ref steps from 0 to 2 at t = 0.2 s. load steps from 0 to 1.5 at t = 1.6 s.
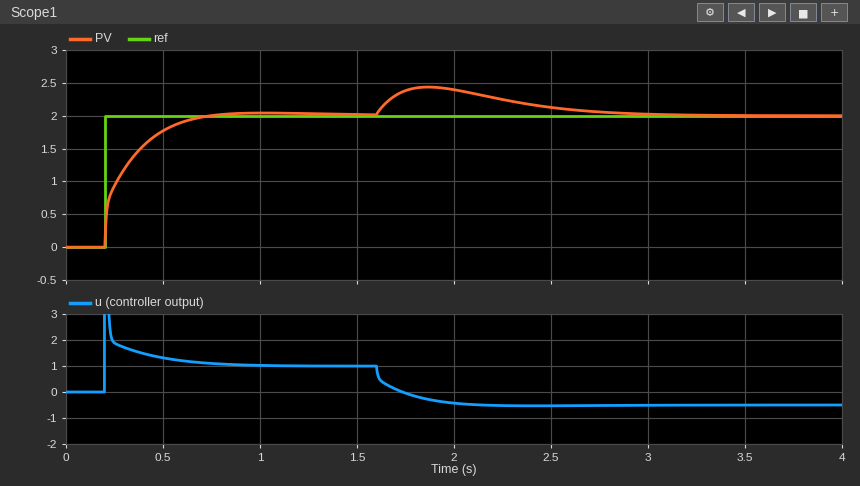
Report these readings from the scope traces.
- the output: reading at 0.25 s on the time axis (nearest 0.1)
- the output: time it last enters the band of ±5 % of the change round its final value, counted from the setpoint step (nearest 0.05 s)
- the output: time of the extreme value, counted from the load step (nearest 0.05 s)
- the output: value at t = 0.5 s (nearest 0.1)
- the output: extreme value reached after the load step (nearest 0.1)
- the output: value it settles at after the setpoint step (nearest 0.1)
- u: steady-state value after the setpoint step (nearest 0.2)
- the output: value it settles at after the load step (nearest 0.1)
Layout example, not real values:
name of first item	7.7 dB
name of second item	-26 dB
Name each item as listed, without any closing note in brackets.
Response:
the output: reading at 0.25 s on the time axis	0.9
the output: time it last enters the band of ±5 % of the change round its final value, counted from the setpoint step	0.40 s
the output: time of the extreme value, counted from the load step	0.25 s
the output: value at t = 0.5 s	1.8
the output: extreme value reached after the load step	2.4
the output: value it settles at after the setpoint step	2.0
u: steady-state value after the setpoint step	1.0
the output: value it settles at after the load step	2.0
